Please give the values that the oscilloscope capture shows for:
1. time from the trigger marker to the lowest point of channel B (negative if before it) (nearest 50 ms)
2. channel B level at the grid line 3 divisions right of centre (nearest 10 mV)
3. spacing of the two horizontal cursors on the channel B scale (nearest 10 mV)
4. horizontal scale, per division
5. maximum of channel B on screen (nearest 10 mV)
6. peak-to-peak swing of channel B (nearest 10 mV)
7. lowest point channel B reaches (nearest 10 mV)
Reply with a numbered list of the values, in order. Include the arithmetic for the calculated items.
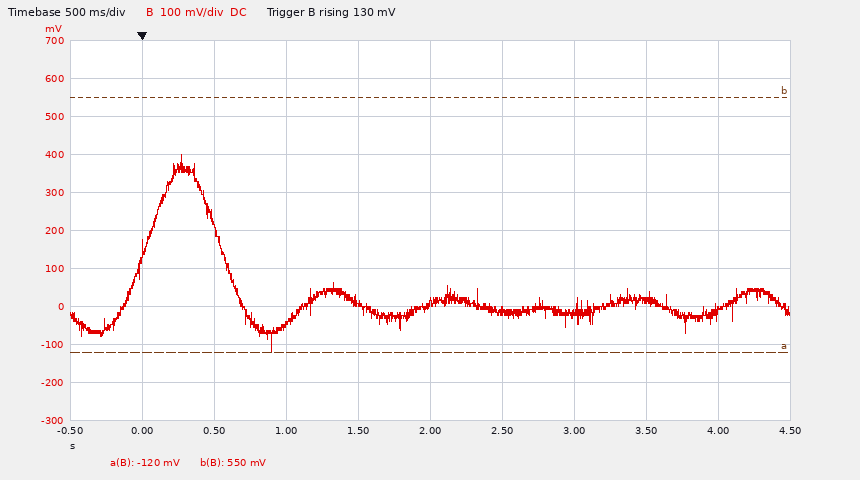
1. +900 ms
2. 20 mV
3. 670 mV
4. 500 ms
5. 400 mV
6. 400 mV − (-120 mV) = 520 mV
7. -120 mV
